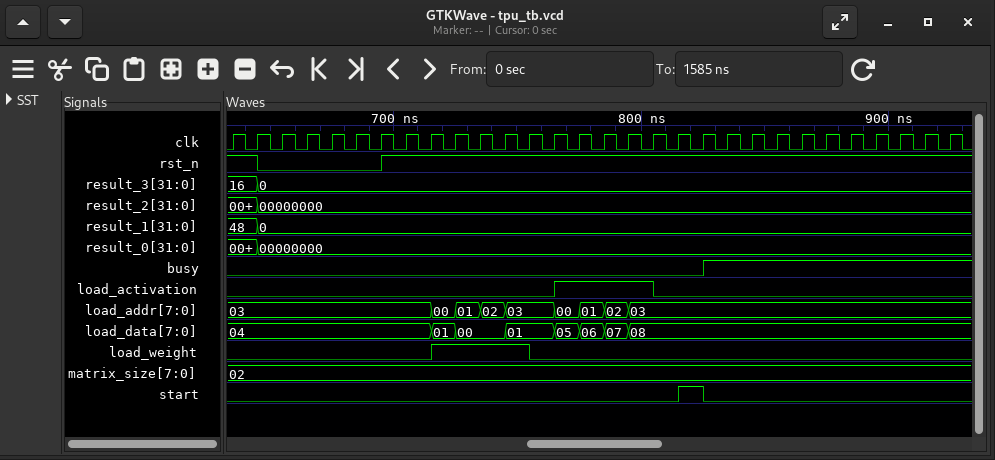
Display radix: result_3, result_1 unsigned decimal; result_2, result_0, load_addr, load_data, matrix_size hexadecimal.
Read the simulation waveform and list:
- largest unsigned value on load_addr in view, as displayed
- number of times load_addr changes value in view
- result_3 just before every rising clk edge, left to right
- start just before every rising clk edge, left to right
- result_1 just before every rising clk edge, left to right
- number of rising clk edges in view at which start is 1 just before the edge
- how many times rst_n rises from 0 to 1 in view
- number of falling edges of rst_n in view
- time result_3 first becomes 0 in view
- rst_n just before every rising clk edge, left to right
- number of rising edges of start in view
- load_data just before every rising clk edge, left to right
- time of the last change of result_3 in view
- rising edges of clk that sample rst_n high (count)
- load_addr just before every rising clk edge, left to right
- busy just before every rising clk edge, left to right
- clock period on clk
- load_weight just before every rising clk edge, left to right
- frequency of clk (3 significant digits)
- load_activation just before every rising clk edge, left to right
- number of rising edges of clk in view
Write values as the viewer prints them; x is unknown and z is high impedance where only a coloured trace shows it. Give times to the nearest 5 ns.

03
8
16, 16, 0, 0, 0, 0, 0, 0, 0, 0, 0, 0, 0, 0, 0, 0, 0, 0, 0, 0, 0, 0, 0, 0, 0, 0, 0, 0, 0, 0
0 0 0 0 0 0 0 0 0 0 0 0 0 0 0 0 0 0 0 1 0 0 0 0 0 0 0 0 0 0
48, 48, 0, 0, 0, 0, 0, 0, 0, 0, 0, 0, 0, 0, 0, 0, 0, 0, 0, 0, 0, 0, 0, 0, 0, 0, 0, 0, 0, 0
1
1
1
645 ns
1 1 0 0 0 0 0 1 1 1 1 1 1 1 1 1 1 1 1 1 1 1 1 1 1 1 1 1 1 1
1
04, 04, 04, 04, 04, 04, 04, 04, 04, 01, 00, 00, 01, 01, 05, 06, 07, 08, 08, 08, 08, 08, 08, 08, 08, 08, 08, 08, 08, 08
645 ns
25
03, 03, 03, 03, 03, 03, 03, 03, 03, 00, 01, 02, 03, 03, 00, 01, 02, 03, 03, 03, 03, 03, 03, 03, 03, 03, 03, 03, 03, 03
0 0 0 0 0 0 0 0 0 0 0 0 0 0 0 0 0 0 0 0 1 1 1 1 1 1 1 1 1 1
10 ns
0 0 0 0 0 0 0 0 0 1 1 1 1 0 0 0 0 0 0 0 0 0 0 0 0 0 0 0 0 0
100 MHz
0 0 0 0 0 0 0 0 0 0 0 0 0 0 1 1 1 1 0 0 0 0 0 0 0 0 0 0 0 0
30
